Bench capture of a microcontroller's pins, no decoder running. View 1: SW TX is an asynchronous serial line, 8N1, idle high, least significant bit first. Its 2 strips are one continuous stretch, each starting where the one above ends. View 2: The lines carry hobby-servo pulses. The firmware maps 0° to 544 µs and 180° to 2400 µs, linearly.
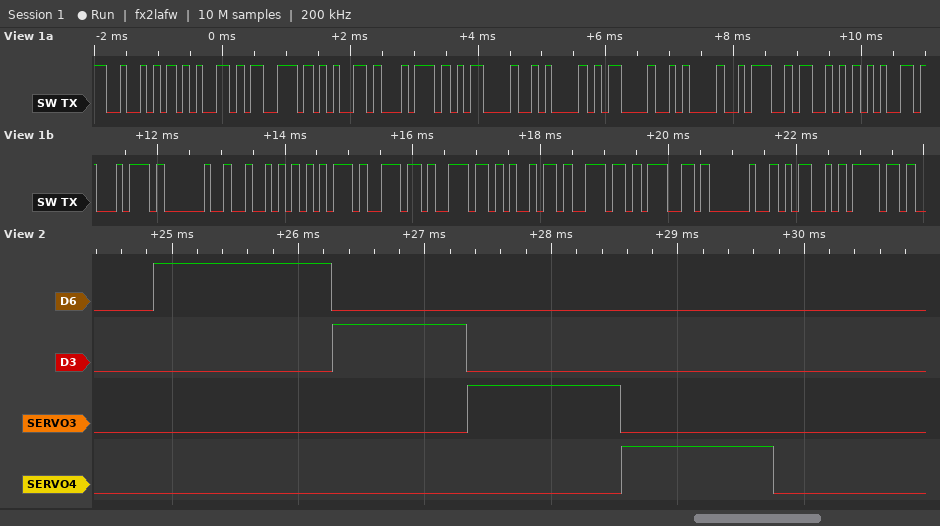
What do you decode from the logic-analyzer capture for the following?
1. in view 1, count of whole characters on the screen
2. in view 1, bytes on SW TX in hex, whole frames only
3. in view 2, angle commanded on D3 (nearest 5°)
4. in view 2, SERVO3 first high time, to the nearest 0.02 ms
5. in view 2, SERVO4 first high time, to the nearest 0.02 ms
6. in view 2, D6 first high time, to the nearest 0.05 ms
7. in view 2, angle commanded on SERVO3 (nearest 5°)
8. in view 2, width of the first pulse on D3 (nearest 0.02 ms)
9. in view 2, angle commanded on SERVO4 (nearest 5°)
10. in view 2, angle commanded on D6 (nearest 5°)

24
52 65 73 65 74 0D 0A 0D 0A 3A 53 65 74 20 52 75 6E 6E 69 6E 67 20 4D 6F
50°
1.20 ms
1.20 ms
1.40 ms
65°
1.06 ms
65°
85°
